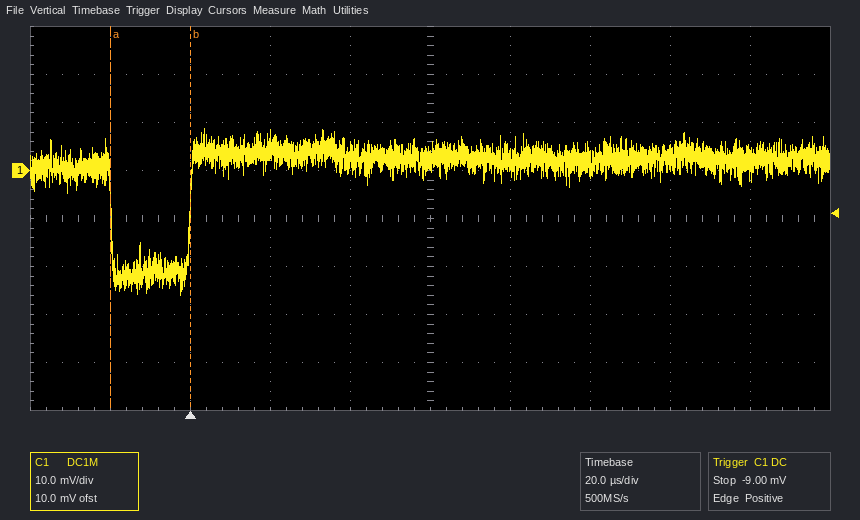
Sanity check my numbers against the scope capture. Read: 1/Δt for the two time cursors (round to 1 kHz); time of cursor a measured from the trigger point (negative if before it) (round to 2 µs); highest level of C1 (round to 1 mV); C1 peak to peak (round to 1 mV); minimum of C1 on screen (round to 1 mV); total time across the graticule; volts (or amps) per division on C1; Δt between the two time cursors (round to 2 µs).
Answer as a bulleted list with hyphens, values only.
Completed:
- 50 kHz
- -20 µs
- 9 mV
- 35 mV
- -26 mV
- 200 µs
- 10 mV
- 20 µs
